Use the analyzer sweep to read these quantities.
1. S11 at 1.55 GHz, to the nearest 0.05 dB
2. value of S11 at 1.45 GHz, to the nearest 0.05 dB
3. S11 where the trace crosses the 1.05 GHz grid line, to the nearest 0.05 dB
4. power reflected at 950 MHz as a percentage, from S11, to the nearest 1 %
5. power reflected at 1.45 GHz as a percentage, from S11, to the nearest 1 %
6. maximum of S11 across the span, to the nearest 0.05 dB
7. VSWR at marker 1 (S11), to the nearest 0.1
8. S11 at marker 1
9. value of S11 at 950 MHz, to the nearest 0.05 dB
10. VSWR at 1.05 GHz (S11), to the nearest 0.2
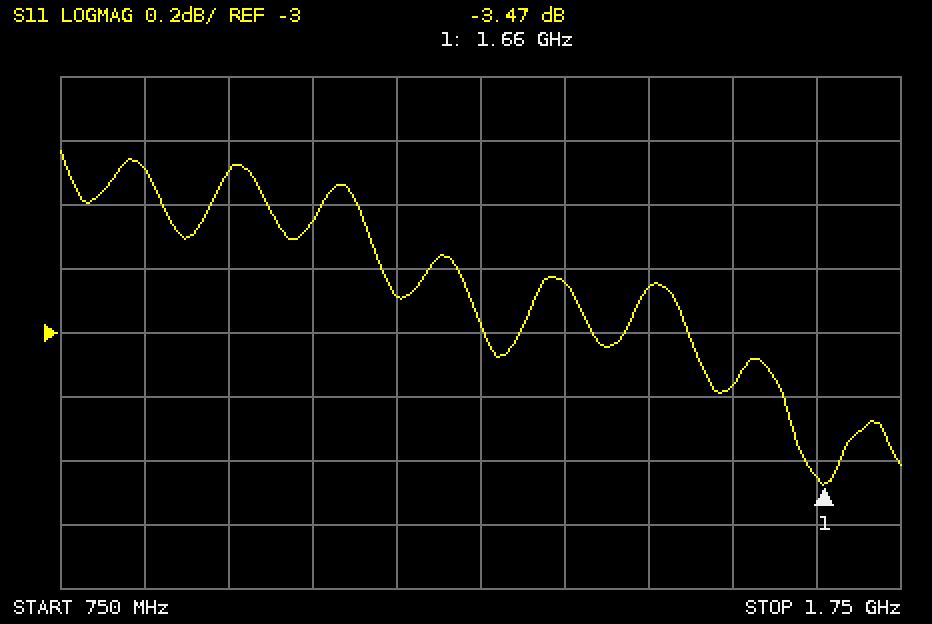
-3.15 dB
-2.85 dB
-2.65 dB
56 %
52 %
-2.45 dB
5.1
-3.47 dB
-2.50 dB
6.6
